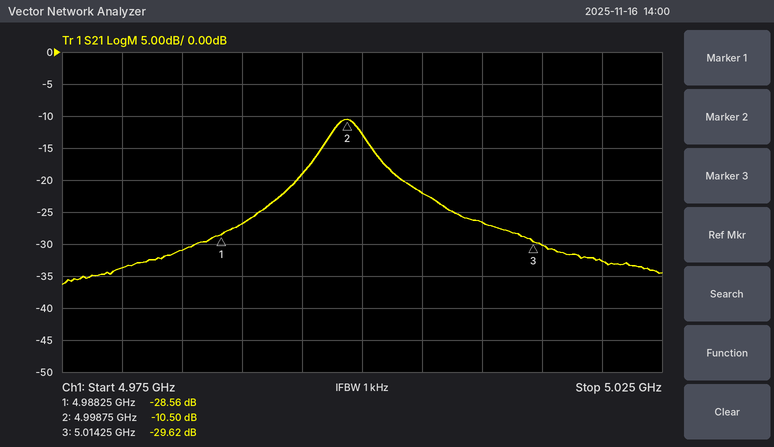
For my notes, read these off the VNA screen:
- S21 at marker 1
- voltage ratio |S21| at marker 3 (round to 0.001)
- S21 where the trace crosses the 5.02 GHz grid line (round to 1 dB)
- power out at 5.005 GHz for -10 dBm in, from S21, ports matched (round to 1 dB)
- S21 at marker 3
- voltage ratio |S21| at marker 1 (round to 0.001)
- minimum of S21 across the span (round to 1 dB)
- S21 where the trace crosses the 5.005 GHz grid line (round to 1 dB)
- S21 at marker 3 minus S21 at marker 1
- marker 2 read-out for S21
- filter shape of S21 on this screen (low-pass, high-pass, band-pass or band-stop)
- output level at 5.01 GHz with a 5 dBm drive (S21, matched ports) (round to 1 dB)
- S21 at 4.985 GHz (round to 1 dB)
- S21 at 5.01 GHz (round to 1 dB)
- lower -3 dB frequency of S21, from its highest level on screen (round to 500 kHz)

-28.56 dB
0.033
-33 dB
-32 dBm
-29.62 dB
0.037
-36 dB
-22 dB
-1.06 dB
-10.50 dB
band-pass
-22 dBm
-31 dB
-27 dB
4.9970 GHz
